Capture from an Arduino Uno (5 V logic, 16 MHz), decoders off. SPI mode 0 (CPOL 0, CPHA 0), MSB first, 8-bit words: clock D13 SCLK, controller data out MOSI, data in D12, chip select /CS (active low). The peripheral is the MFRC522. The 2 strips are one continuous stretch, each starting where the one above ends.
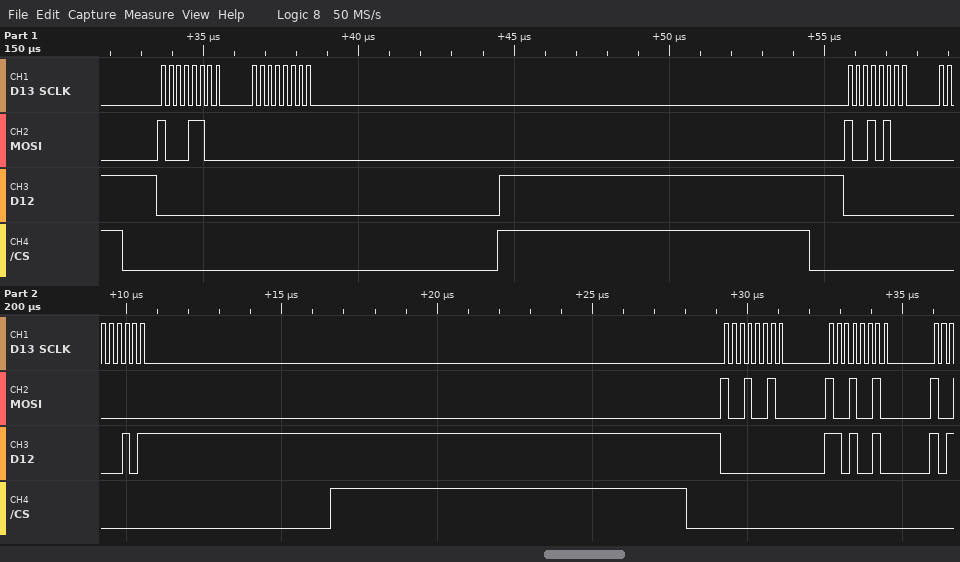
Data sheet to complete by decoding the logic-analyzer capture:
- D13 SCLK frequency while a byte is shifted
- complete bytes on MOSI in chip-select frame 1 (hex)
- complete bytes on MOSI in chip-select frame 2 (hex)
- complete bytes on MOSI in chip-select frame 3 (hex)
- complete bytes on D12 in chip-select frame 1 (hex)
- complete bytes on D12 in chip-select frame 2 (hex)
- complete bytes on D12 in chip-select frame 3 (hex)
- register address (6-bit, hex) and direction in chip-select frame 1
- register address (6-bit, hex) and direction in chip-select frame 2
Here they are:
4 MHz
8C 00
94 00
92 92
00 00
00 05
00 D2
0x06 read
0x0A read
